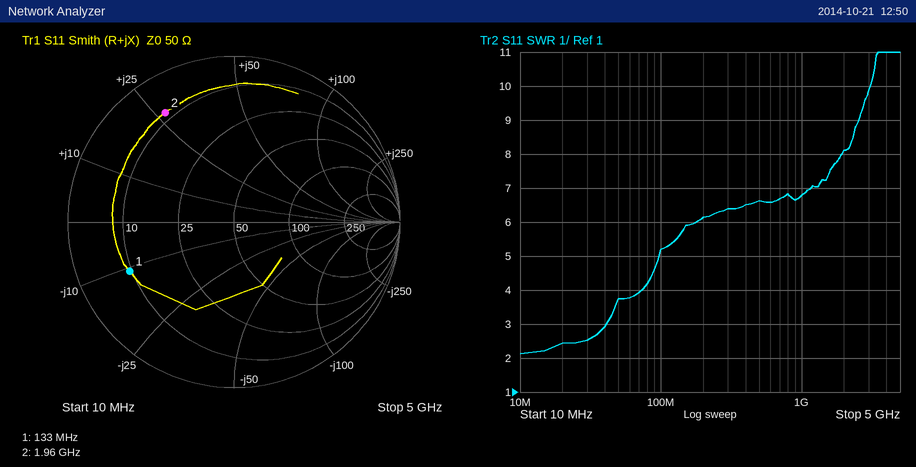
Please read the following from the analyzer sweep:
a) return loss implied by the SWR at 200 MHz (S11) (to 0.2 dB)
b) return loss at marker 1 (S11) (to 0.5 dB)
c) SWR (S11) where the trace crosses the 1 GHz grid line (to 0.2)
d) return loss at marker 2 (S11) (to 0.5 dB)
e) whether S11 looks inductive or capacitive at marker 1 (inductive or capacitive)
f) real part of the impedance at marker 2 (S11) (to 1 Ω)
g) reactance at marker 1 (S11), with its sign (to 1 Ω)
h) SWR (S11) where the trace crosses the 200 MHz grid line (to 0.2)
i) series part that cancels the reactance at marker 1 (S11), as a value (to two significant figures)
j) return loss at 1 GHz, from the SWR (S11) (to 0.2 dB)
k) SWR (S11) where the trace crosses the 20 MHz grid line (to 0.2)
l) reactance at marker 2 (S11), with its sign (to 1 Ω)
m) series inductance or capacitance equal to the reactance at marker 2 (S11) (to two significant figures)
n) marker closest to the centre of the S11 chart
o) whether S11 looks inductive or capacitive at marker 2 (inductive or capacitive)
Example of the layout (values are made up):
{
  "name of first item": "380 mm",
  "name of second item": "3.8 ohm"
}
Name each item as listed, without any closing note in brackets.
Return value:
{
  "return loss implied by the SWR at 200 MHz (S11)": "2.8 dB",
  "return loss at marker 1 (S11)": "3.0 dB",
  "SWR (S11) where the trace crosses the 1 GHz grid line": "6.8",
  "return loss at marker 2 (S11)": "2.0 dB",
  "whether S11 looks inductive or capacitive at marker 1": "capacitive",
  "real part of the impedance at marker 2 (S11)": "8 Ω",
  "reactance at marker 1 (S11), with its sign": "-11 Ω",
  "SWR (S11) where the trace crosses the 200 MHz grid line": "6.2",
  "series part that cancels the reactance at marker 1 (S11), as a value": "13 nH",
  "return loss at 1 GHz, from the SWR (S11)": "2.6 dB",
  "SWR (S11) where the trace crosses the 20 MHz grid line": "2.4",
  "reactance at marker 2 (S11), with its sign": "+27 Ω",
  "series inductance or capacitance equal to the reactance at marker 2 (S11)": "2.2 nH",
  "marker closest to the centre of the S11 chart": "marker 1",
  "whether S11 looks inductive or capacitive at marker 2": "inductive"
}
